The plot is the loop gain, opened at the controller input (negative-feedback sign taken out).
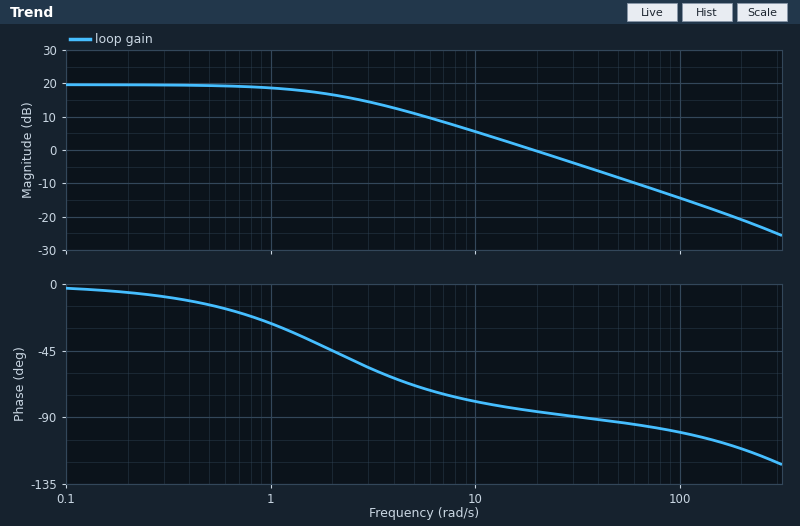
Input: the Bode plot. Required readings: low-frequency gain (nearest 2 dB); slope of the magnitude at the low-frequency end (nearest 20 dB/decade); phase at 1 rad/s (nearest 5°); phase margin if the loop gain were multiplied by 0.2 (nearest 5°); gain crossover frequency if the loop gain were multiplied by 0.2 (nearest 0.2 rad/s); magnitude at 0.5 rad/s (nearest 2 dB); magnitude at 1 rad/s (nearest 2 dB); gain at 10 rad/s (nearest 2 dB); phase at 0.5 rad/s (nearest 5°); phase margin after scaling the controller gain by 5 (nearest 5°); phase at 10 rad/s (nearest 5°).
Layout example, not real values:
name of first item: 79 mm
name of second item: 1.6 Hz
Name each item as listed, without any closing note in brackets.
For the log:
low-frequency gain: 20 dB
slope of the magnitude at the low-frequency end: 0 dB/decade
phase at 1 rad/s: -25°
phase margin if the loop gain were multiplied by 0.2: 120°
gain crossover frequency if the loop gain were multiplied by 0.2: 3.2 rad/s
magnitude at 0.5 rad/s: 20 dB
magnitude at 1 rad/s: 18 dB
gain at 10 rad/s: 6 dB
phase at 0.5 rad/s: -15°
phase margin after scaling the controller gain by 5: 80°
phase at 10 rad/s: -80°
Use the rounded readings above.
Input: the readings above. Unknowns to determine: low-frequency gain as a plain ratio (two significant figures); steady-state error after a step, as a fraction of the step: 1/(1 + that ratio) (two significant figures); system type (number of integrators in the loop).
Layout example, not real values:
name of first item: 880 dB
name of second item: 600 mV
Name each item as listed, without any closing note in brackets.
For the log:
low-frequency gain as a plain ratio: 10
steady-state error after a step, as a fraction of the step: 1/(1 + that ratio): 0.091
system type: 0
